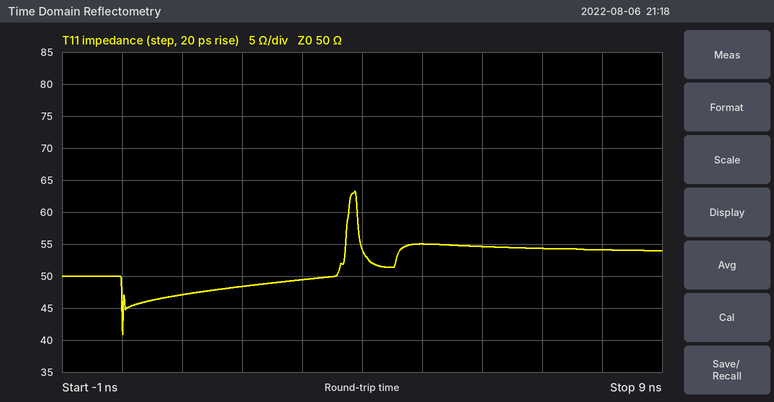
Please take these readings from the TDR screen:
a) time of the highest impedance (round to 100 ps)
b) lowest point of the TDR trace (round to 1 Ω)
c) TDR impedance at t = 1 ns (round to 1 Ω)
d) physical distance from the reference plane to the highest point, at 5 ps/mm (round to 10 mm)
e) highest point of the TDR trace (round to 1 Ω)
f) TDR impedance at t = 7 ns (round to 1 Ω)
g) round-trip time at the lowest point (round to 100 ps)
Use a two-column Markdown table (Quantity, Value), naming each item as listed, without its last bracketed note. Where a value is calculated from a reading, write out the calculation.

| Quantity | Value |
|---|---|
| time of the highest impedance | 3.9 ns |
| lowest point of the TDR trace | 41 Ω |
| TDR impedance at t = 1 ns | 47 Ω |
| physical distance from the reference plane to the highest point, at 5 ps/mm | 3.9 ns / 2 / 5 ps/mm ≈ 390 mm |
| highest point of the TDR trace | 63 Ω |
| TDR impedance at t = 7 ns | 54 Ω |
| round-trip time at the lowest point | 0.0 ns |
